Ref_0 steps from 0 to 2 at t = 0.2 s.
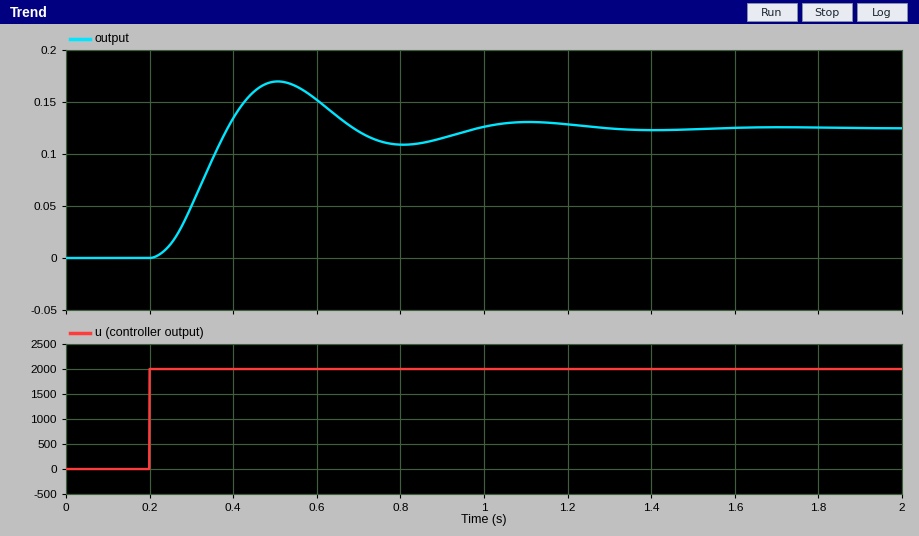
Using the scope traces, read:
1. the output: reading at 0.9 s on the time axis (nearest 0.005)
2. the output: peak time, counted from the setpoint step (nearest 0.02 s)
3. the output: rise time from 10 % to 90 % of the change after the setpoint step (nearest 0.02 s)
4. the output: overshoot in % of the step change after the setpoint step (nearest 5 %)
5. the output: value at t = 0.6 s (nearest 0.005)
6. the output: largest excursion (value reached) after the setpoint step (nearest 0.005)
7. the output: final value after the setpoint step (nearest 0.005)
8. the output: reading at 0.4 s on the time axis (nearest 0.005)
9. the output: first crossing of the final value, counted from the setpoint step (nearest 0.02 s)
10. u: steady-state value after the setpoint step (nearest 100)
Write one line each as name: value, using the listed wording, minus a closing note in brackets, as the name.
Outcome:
the output: reading at 0.9 s on the time axis: 0.115
the output: peak time, counted from the setpoint step: 0.30 s
the output: rise time from 10 % to 90 % of the change after the setpoint step: 0.12 s
the output: overshoot in % of the step change after the setpoint step: 35 %
the output: value at t = 0.6 s: 0.150
the output: largest excursion (value reached) after the setpoint step: 0.170
the output: final value after the setpoint step: 0.125
the output: reading at 0.4 s on the time axis: 0.135
the output: first crossing of the final value, counted from the setpoint step: 0.18 s
u: steady-state value after the setpoint step: 2000
